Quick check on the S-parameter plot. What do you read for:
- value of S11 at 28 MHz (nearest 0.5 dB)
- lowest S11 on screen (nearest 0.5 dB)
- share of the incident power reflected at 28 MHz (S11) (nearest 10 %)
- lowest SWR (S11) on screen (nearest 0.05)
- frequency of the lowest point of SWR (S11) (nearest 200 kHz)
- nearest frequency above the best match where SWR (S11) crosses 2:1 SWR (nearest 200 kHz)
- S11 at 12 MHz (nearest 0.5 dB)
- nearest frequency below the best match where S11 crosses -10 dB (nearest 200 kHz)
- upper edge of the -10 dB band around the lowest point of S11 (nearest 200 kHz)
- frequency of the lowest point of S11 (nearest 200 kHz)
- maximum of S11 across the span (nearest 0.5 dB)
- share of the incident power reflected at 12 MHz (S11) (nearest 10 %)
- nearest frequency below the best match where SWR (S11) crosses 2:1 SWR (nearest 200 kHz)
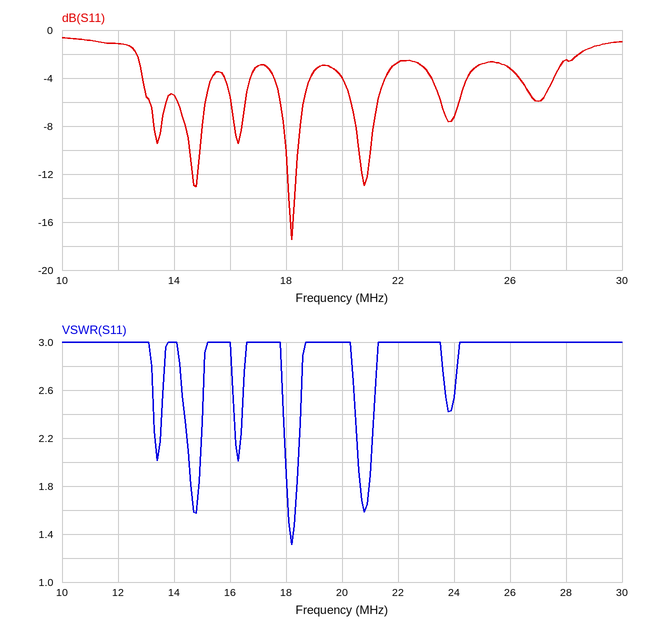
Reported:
-2.5 dB
-17.5 dB
60 %
1.30
18.2 MHz
18.4 MHz
-1.0 dB
18.0 MHz
18.4 MHz
18.2 MHz
-0.5 dB
80 %
18.0 MHz
